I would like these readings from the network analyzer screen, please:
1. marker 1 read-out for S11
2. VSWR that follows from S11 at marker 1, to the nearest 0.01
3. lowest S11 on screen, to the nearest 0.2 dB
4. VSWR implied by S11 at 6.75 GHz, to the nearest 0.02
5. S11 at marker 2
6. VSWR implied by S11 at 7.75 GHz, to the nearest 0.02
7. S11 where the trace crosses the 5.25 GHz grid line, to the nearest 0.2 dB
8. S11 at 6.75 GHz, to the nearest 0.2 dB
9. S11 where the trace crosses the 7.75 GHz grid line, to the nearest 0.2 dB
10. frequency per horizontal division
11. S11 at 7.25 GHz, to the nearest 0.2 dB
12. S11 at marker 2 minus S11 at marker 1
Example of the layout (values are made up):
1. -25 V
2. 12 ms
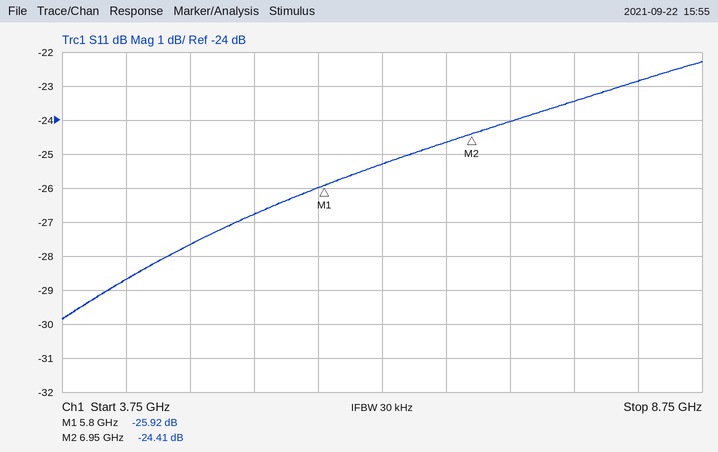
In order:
1. -25.92 dB
2. 1.11
3. -29.8 dB
4. 1.12
5. -24.41 dB
6. 1.14
7. -26.8 dB
8. -24.6 dB
9. -23.4 dB
10. 500 MHz
11. -24.0 dB
12. 1.51 dB
